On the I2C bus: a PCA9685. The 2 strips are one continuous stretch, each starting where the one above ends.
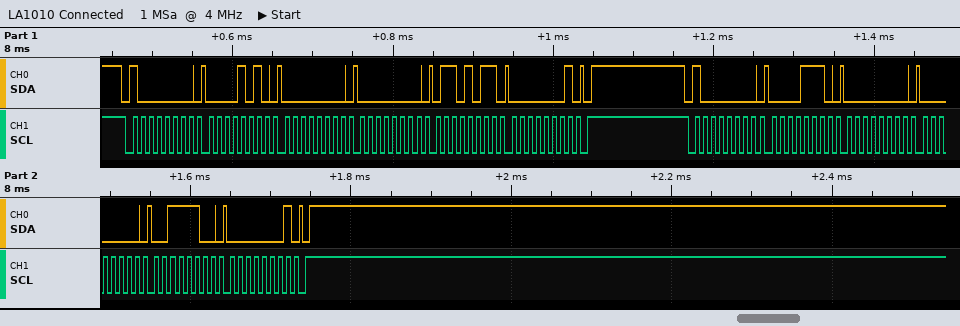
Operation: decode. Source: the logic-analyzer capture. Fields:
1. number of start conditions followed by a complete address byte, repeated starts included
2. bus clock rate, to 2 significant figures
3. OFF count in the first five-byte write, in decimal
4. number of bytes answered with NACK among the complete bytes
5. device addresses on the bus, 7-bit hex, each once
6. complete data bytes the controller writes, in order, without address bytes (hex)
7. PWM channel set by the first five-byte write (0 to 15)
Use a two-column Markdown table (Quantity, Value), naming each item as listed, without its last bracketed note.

| Quantity | Value |
|---|---|
| number of start conditions followed by a complete address byte, repeated starts included | 2 |
| bus clock rate, to 2 significant figures | 100 kHz |
| OFF count in the first five-byte write, in decimal | 363 |
| number of bytes answered with NACK among the complete bytes | 0 |
| device addresses on the bus, 7-bit hex, each once | 0x40 |
| complete data bytes the controller writes, in order, without address bytes | 0A 00 00 6B 01 0E 00 00 3C 01 |
| PWM channel set by the first five-byte write | 1 |
